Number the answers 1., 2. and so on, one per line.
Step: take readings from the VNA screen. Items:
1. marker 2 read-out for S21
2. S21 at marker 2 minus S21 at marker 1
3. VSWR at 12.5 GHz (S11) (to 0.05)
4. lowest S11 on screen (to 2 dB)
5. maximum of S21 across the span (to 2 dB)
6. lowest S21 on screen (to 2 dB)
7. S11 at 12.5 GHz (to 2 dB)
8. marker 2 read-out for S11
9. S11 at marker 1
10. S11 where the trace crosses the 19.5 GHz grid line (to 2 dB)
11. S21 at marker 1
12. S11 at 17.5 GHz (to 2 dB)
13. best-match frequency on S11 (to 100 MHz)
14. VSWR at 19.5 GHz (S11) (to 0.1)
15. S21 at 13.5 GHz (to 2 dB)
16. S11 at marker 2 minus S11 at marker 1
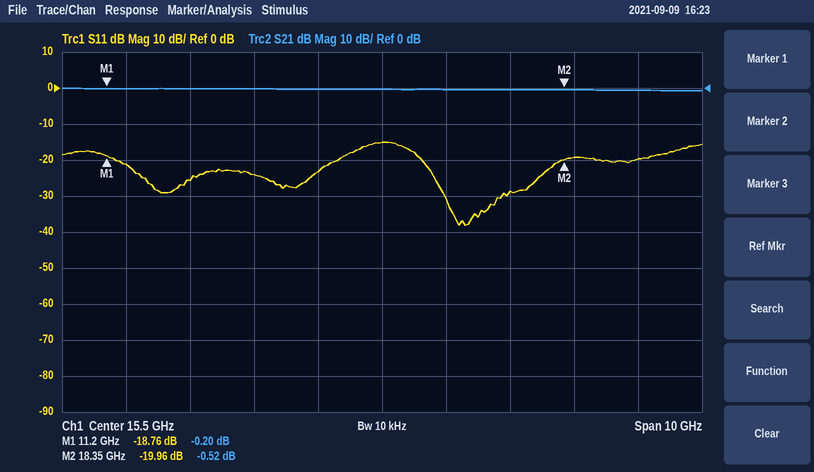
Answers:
1. -0.52 dB
2. -0.32 dB
3. 1.10
4. -38 dB
5. 0 dB
6. 0 dB
7. -26 dB
8. -19.96 dB
9. -18.76 dB
10. -20 dB
11. -0.20 dB
12. -28 dB
13. 16.8 GHz
14. 1.2
15. 0 dB
16. -1.20 dB
